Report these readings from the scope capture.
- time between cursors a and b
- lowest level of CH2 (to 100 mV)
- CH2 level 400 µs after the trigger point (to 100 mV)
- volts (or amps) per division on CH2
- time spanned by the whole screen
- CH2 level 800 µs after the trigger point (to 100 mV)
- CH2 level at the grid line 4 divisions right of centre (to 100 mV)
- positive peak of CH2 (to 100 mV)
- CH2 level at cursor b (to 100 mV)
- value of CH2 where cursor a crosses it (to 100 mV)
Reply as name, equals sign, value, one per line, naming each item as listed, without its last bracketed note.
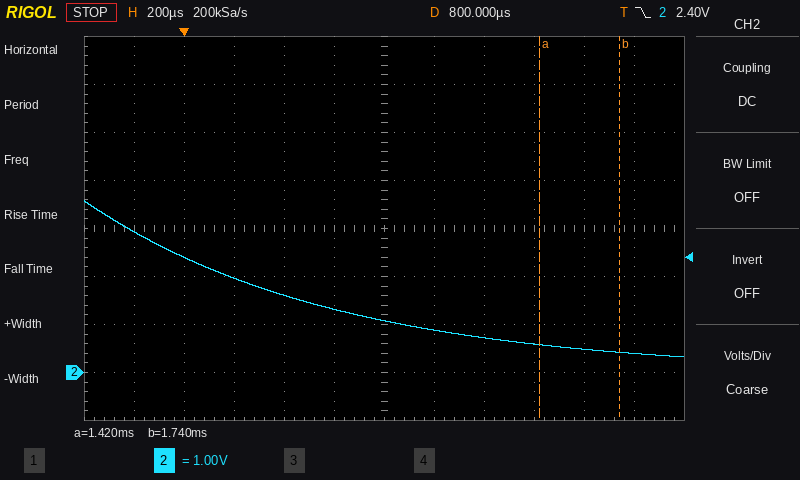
time between cursors a and b = 320 µs
lowest level of CH2 = 300 mV
CH2 level 400 µs after the trigger point = 1.6 V
volts (or amps) per division on CH2 = 1 V
time spanned by the whole screen = 2.4 ms
CH2 level 800 µs after the trigger point = 1.1 V
CH2 level at the grid line 4 divisions right of centre = 500 mV
positive peak of CH2 = 3.6 V
CH2 level at cursor b = 400 mV
value of CH2 where cursor a crosses it = 600 mV
